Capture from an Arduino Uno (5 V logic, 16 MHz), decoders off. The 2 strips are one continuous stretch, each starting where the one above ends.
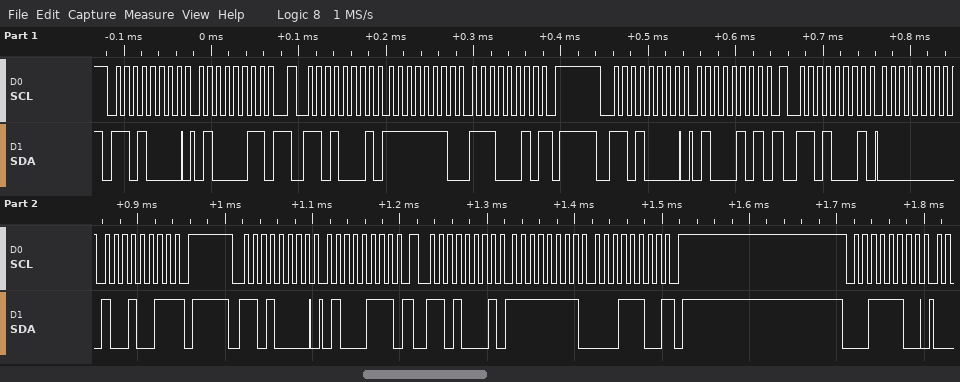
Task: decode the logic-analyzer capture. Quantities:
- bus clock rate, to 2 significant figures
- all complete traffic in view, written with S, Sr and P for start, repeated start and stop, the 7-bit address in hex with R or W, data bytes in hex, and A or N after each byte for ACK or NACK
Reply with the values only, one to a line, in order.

100 kHz
S 68W A 43 A Sr 68R A FE A E2 N P S 68W A 45 A Sr 68R A 00 A 93 N P S 68W A 47 A Sr 68R A FF A 1C N P S 1EW A
